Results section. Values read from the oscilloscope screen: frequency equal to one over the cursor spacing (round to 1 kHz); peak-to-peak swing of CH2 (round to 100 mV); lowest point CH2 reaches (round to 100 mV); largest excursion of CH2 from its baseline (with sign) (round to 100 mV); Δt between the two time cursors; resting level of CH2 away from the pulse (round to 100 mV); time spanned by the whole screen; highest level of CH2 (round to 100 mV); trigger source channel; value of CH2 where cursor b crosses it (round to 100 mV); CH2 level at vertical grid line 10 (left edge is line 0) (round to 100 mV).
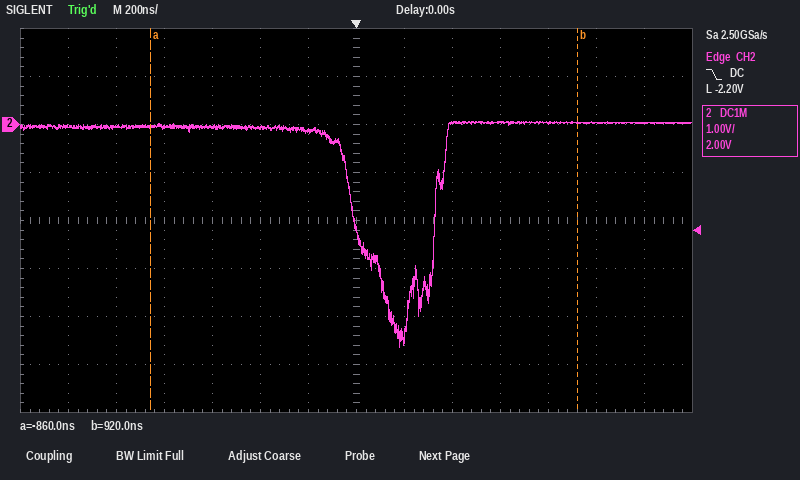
562 kHz
4.7 V
-4.6 V
-4.6 V
1.78 µs
0.0 V
2.8 µs
100 mV
CH2
0.0 V
0.0 V
